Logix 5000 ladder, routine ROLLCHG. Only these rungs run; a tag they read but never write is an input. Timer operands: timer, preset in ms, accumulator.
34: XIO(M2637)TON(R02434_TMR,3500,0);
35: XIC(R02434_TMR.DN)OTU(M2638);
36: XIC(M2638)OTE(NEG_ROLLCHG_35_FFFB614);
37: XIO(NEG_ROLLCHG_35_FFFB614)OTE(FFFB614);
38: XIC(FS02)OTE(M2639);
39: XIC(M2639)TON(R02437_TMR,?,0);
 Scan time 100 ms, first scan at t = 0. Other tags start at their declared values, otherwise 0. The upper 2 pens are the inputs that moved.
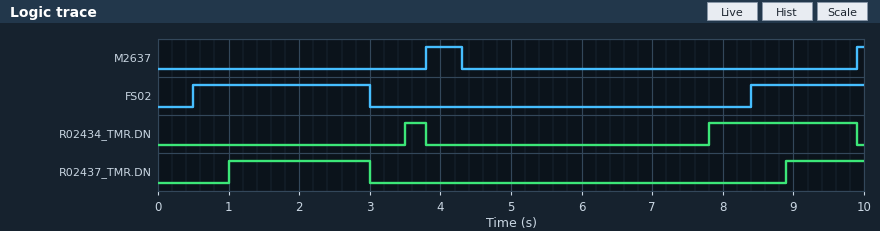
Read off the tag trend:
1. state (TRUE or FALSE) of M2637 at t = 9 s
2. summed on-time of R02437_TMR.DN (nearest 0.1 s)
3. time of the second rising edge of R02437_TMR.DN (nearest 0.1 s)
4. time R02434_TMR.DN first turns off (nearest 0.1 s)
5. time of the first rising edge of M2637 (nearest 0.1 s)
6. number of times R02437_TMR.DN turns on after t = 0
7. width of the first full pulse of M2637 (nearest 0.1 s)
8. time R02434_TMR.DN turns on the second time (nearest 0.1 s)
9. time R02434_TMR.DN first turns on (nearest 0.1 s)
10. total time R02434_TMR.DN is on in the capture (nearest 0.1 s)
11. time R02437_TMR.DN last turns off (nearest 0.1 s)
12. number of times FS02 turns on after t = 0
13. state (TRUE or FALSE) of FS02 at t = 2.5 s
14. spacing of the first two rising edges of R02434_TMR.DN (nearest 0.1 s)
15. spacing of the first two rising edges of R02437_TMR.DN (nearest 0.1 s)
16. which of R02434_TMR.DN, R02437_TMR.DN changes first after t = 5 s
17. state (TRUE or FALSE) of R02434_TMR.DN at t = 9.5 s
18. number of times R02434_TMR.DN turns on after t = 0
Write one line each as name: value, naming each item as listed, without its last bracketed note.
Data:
state (TRUE or FALSE) of M2637 at t = 9 s: FALSE
summed on-time of R02437_TMR.DN: 3.1 s
time of the second rising edge of R02437_TMR.DN: 8.9 s
time R02434_TMR.DN first turns off: 3.8 s
time of the first rising edge of M2637: 3.8 s
number of times R02437_TMR.DN turns on after t = 0: 2
width of the first full pulse of M2637: 0.5 s
time R02434_TMR.DN turns on the second time: 7.8 s
time R02434_TMR.DN first turns on: 3.5 s
total time R02434_TMR.DN is on in the capture: 2.4 s
time R02437_TMR.DN last turns off: 3.0 s
number of times FS02 turns on after t = 0: 2
state (TRUE or FALSE) of FS02 at t = 2.5 s: TRUE
spacing of the first two rising edges of R02434_TMR.DN: 4.3 s
spacing of the first two rising edges of R02437_TMR.DN: 7.9 s
which of R02434_TMR.DN, R02437_TMR.DN changes first after t = 5 s: R02434_TMR.DN
state (TRUE or FALSE) of R02434_TMR.DN at t = 9.5 s: TRUE
number of times R02434_TMR.DN turns on after t = 0: 2
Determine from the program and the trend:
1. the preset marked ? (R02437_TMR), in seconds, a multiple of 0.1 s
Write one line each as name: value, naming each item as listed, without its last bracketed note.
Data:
the preset marked ? (R02437_TMR), in seconds, a multiple of 0.1 s: 0.5 s
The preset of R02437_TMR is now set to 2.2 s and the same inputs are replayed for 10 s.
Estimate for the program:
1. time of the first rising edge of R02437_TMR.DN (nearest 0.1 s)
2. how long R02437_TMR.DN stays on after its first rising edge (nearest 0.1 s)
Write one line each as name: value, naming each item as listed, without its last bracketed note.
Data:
time of the first rising edge of R02437_TMR.DN: 2.7 s
how long R02437_TMR.DN stays on after its first rising edge: 0.3 s
